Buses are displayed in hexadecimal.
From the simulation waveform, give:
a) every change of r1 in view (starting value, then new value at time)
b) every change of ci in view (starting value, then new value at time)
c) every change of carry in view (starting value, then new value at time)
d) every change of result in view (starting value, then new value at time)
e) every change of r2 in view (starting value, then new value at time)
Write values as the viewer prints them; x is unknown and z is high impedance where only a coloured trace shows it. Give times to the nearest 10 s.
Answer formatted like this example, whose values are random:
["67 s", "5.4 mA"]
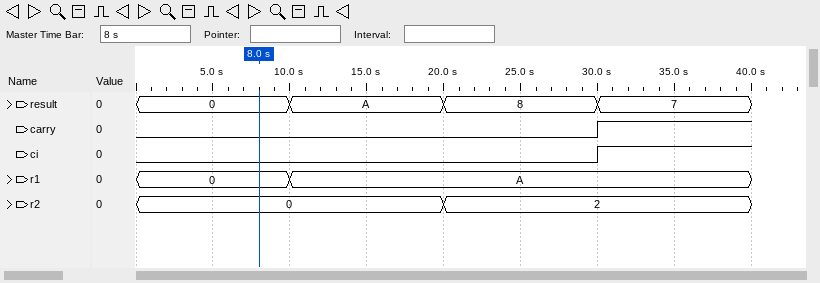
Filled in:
["0, A at 10 s", "0, 1 at 30 s", "0, 1 at 30 s", "0, A at 10 s, 8 at 20 s, 7 at 30 s", "0, 2 at 20 s"]
